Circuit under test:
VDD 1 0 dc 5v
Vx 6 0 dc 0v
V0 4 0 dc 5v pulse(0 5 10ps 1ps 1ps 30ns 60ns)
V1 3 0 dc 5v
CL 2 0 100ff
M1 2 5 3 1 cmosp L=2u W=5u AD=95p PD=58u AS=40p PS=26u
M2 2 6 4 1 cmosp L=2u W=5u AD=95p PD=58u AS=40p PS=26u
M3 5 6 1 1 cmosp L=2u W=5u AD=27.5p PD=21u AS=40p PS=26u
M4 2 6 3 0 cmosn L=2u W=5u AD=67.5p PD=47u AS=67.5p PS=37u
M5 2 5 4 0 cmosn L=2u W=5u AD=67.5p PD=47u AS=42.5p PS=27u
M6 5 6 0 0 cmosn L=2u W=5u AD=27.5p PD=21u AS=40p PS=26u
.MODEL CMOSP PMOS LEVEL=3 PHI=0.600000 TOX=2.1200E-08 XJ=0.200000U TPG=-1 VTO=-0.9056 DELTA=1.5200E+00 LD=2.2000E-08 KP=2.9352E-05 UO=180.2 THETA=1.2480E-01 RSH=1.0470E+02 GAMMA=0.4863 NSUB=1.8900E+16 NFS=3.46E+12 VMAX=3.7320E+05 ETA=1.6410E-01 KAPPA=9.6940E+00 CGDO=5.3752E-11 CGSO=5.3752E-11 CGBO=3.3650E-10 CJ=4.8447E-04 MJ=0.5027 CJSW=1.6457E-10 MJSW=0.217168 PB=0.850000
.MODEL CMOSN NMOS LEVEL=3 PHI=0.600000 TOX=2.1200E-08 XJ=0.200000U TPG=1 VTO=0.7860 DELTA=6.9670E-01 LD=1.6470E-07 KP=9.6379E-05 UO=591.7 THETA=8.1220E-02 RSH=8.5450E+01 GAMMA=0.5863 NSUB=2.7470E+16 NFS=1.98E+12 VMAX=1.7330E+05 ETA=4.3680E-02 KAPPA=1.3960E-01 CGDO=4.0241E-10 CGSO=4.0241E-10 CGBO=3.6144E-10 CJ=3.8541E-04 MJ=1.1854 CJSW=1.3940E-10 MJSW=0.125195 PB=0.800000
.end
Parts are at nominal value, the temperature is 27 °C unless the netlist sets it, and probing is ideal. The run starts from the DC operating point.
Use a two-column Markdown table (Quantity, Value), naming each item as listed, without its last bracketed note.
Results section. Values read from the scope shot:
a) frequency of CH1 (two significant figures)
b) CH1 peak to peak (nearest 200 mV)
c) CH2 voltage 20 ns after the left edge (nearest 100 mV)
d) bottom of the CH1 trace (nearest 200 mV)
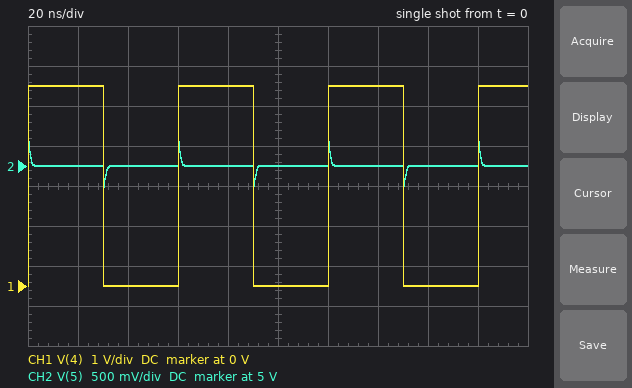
| Quantity | Value |
|---|---|
| frequency of CH1 | 17 MHz |
| CH1 peak to peak | 5.0 V |
| CH2 voltage 20 ns after the left edge | 5.0 V |
| bottom of the CH1 trace | 0 V |
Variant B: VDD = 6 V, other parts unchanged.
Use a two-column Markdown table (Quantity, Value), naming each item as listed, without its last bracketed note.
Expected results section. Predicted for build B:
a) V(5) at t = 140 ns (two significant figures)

| Quantity | Value |
|---|---|
| V(5) at t = 140 ns | 6.0 V |
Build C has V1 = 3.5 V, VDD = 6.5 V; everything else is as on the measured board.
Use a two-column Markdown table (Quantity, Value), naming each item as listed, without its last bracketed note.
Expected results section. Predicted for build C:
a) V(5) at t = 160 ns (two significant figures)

| Quantity | Value |
|---|---|
| V(5) at t = 160 ns | 6.5 V |
